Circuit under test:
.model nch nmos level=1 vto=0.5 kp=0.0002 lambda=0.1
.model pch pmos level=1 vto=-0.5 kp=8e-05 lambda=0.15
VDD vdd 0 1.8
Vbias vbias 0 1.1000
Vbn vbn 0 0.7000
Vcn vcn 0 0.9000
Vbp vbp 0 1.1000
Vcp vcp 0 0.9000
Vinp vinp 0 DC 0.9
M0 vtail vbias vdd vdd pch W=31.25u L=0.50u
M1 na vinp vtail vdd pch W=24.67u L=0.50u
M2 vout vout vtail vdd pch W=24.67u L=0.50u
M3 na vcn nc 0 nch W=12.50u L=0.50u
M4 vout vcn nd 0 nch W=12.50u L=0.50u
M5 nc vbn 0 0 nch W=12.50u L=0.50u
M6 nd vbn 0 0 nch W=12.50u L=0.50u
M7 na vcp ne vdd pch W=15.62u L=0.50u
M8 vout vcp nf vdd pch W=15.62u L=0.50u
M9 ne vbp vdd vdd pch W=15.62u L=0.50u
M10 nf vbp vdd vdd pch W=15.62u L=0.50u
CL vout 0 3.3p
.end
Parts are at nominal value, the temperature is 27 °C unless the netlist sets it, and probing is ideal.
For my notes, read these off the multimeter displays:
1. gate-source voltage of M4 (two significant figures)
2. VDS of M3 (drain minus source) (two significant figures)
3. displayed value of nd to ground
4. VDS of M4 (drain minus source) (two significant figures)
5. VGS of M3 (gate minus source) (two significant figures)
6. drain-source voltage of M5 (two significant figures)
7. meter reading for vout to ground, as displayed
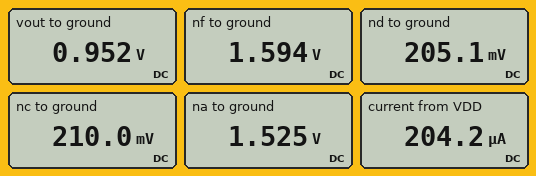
690 mV
1.3 V
205.1 mV
750 mV
690 mV
210 mV
0.952 V
